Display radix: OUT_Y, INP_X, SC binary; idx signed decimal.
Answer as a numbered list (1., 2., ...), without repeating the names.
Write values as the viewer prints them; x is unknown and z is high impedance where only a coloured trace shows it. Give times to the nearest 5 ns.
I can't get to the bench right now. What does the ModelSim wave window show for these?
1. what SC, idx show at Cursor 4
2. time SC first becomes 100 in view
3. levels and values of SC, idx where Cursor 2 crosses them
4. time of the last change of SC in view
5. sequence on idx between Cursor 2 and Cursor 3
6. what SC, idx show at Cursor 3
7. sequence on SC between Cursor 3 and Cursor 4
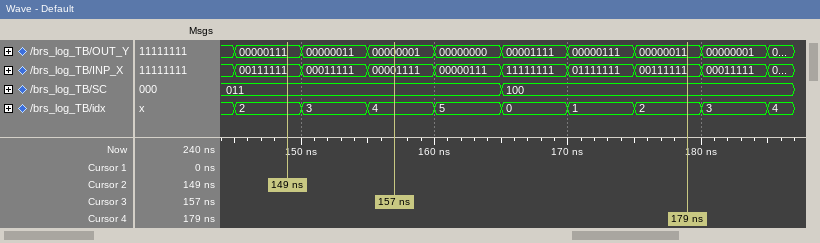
1. SC=100, idx=2
2. 165 ns
3. SC=011, idx=2
4. 165 ns
5. 2, 3, 4
6. SC=011, idx=4
7. 011, 100
